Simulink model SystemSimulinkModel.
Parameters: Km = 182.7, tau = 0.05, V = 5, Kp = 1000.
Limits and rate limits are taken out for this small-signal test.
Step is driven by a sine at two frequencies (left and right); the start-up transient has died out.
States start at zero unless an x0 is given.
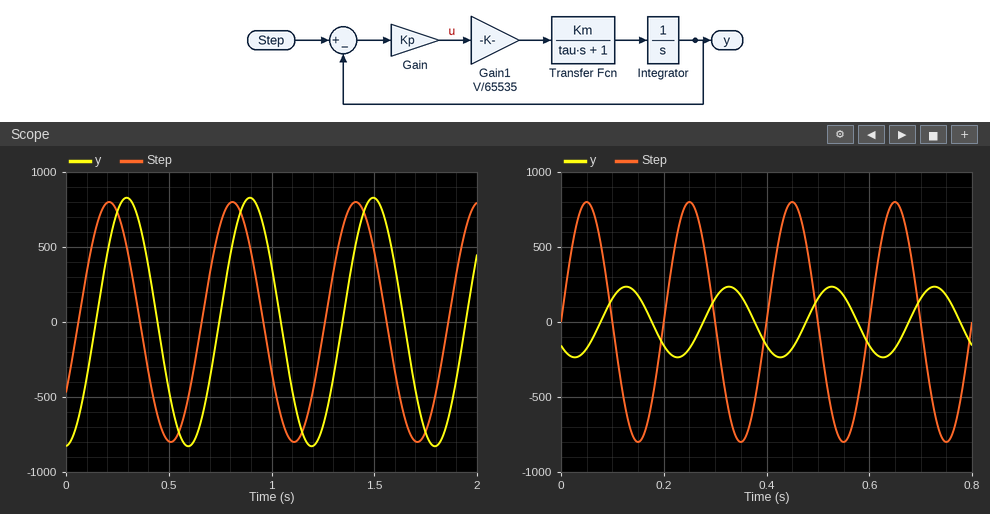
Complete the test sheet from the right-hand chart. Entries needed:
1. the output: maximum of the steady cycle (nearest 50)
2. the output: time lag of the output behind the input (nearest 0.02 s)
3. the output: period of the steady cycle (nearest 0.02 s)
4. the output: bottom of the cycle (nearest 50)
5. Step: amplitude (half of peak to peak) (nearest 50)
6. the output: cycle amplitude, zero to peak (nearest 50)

250
0.08 s
0.20 s
-250
800
250
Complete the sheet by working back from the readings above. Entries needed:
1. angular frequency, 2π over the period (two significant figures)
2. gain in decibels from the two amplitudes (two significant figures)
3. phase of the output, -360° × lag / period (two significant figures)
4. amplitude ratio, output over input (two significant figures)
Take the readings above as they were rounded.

31 rad/s
-10 dB
-140°
0.31
